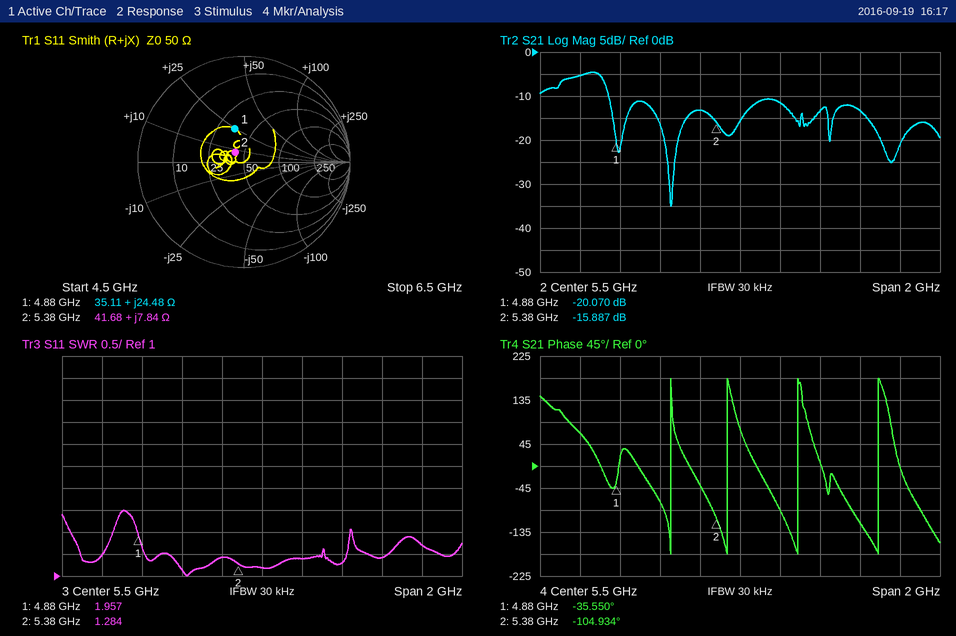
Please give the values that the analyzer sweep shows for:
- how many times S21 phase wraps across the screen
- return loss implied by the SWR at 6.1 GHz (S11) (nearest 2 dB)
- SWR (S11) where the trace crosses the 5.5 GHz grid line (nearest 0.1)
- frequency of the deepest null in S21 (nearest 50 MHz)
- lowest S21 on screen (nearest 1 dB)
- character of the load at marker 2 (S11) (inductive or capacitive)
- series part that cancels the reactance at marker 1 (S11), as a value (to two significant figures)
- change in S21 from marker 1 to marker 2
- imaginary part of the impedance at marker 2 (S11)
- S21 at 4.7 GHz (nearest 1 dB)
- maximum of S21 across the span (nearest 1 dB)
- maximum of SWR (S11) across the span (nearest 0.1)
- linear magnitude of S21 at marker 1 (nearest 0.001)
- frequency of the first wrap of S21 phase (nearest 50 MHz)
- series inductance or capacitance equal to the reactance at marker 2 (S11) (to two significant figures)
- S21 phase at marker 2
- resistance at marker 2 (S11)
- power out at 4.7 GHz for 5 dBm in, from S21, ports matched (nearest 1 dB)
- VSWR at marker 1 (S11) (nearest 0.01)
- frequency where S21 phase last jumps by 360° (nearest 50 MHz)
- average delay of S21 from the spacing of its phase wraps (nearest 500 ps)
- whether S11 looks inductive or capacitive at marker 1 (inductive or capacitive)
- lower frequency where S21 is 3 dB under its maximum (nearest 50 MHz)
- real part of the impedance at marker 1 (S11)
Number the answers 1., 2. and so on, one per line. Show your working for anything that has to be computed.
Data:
1. 4
2. −20 log10((1.4 − 1)/(1.4 + 1)) ≈ 16 dB
3. 1.2
4. 5.15 GHz
5. -35 dB
6. inductive
7. C = 1/(2π × 4.88 GHz × 24.48 Ω) ≈ 1.3 pF
8. -15.887 − (-20.07) = 4.183 dB
9. +7.84 Ω
10. -5 dB
11. -5 dB
12. 2.5
13. 10^(-20.07/20) ≈ 0.099
14. 5.15 GHz
15. L = 7.84 Ω/(2π × 5.38 GHz) ≈ 232 pH, so 230 pH to two significant figures
16. -104.934°
17. 41.68 Ω
18. 5 dBm + (-5 dB) = 0 dBm
19. 1.96
20. 6.20 GHz
21. 3 cycles / (6.20 GHz − 5.15 GHz) ≈ 2.86 ns, so 3.0 ns to the nearest 500 ps
22. inductive
23. 4.60 GHz
24. 35.11 Ω
